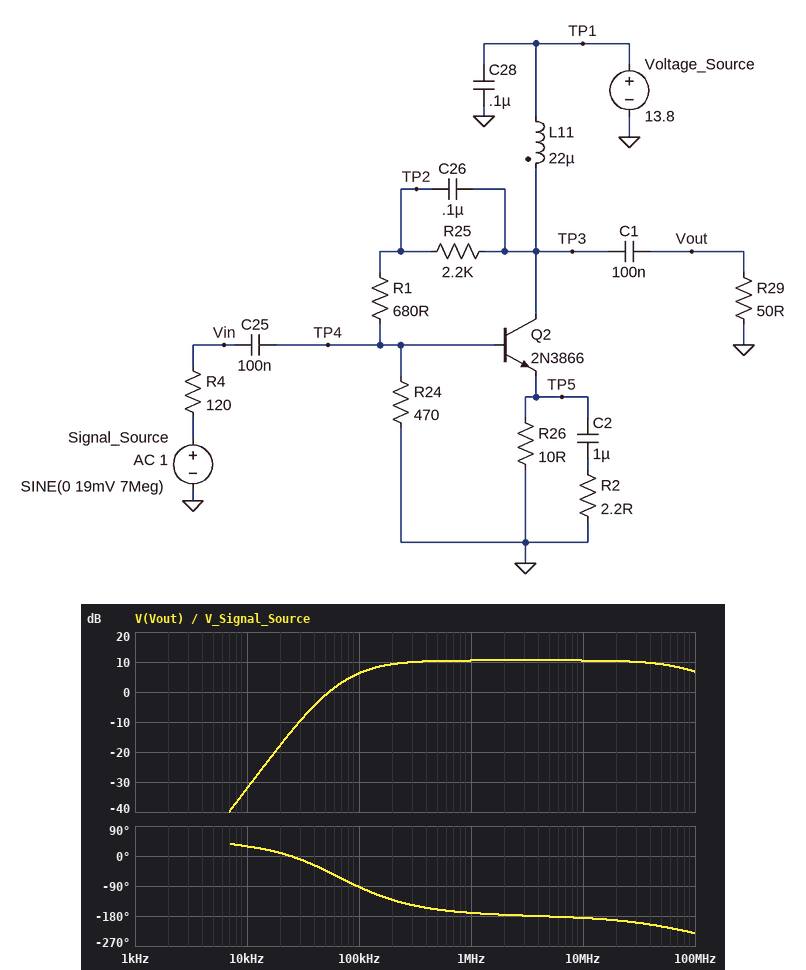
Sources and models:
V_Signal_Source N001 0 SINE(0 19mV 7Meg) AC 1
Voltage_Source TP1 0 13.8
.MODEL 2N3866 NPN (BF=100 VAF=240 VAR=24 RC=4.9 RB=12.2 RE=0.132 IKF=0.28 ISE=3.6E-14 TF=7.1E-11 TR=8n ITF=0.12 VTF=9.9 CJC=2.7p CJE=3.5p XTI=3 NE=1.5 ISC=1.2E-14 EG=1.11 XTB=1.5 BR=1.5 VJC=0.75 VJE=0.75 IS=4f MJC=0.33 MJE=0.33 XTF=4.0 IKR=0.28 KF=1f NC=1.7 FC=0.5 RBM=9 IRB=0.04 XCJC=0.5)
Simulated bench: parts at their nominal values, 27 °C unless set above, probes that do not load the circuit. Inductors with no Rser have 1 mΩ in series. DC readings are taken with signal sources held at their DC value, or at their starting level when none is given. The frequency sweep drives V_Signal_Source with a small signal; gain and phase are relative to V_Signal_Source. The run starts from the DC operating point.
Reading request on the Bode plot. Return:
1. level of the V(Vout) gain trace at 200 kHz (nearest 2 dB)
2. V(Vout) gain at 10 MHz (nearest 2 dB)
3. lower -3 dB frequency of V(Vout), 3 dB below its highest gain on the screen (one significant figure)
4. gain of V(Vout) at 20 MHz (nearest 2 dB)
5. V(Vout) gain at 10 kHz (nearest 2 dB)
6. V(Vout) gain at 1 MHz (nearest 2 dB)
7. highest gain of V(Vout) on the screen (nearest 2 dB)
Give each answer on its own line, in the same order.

10 dB
10 dB
100 kHz
10 dB
-32 dB
10 dB
10 dB
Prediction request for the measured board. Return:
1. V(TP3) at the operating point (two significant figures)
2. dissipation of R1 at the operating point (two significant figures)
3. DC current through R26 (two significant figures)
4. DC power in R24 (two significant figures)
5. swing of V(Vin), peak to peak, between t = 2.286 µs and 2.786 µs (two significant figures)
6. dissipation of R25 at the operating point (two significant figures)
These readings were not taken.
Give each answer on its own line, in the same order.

14 V
12 mW
74 mA
5.2 mW
7.1 mV
40 mW
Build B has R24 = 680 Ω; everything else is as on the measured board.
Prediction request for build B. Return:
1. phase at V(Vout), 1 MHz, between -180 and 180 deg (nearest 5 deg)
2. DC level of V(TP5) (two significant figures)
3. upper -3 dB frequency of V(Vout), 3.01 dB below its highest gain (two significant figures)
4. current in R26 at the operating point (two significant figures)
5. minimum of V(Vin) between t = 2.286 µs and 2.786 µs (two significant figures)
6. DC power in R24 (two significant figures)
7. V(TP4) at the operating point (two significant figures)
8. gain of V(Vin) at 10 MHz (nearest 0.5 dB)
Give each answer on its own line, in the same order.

-170 deg
1.0 V
73 MHz
100 mA
-3.4 mV
5.1 mW
1.9 V
-15.0 dB
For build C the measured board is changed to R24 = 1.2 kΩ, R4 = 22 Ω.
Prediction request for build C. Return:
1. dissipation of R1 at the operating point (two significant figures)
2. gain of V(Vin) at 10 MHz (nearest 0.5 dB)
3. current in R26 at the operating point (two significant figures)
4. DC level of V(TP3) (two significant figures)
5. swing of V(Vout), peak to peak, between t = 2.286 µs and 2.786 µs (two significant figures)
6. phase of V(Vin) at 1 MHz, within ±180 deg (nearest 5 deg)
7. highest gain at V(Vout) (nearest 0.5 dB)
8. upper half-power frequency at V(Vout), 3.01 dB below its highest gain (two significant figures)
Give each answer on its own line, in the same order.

11 mW
-5.5 dB
140 mA
14 V
390 mV
-10 deg
20.0 dB
80 MHz
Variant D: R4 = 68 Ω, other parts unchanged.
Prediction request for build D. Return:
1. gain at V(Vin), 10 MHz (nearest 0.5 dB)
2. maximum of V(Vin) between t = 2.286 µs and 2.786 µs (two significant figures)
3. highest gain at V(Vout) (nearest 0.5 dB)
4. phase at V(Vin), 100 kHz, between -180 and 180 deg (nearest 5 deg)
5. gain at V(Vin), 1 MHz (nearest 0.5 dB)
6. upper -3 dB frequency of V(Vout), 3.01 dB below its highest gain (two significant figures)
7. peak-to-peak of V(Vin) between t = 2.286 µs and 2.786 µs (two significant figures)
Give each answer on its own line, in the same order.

-11.0 dB
5.5 mV
14.5 dB
-25 deg
-10.5 dB
91 MHz
11 mV
